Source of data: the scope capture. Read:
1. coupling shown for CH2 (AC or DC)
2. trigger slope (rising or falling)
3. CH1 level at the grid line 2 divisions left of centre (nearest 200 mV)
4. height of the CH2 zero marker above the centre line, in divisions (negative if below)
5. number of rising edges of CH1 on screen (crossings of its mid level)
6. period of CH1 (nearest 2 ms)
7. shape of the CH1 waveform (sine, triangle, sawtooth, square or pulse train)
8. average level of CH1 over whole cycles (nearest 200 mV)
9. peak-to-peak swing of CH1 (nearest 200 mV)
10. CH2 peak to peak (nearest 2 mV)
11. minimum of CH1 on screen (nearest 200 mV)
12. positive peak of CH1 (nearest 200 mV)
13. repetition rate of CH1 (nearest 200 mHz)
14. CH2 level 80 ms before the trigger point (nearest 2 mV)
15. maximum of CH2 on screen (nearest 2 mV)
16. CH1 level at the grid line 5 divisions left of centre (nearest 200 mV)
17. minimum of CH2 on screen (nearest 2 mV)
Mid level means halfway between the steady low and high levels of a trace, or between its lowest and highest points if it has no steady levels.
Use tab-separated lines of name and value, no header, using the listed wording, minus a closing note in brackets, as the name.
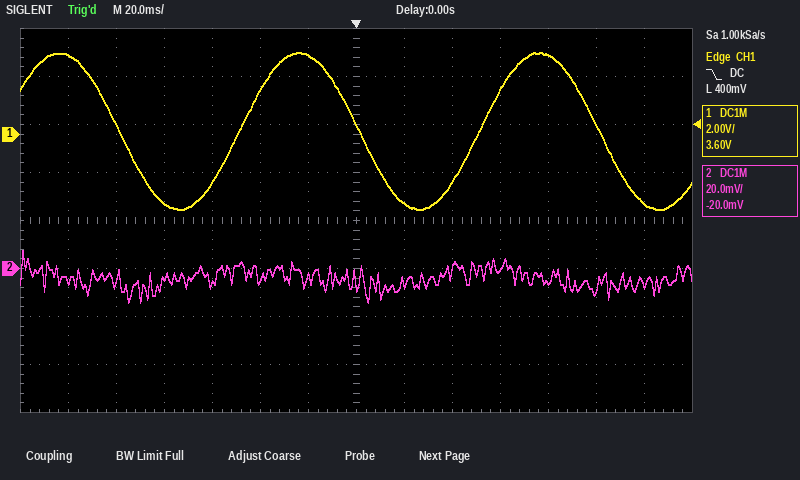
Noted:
coupling shown for CH2	DC
trigger slope	falling
CH1 level at the grid line 2 divisions left of centre	1.8 V
height of the CH2 zero marker above the centre line, in divisions	-1.0 div
number of rising edges of CH1 on screen	2
period of CH1	100 ms
shape of the CH1 waveform	sine
average level of CH1 over whole cycles	200 mV
peak-to-peak swing of CH1	6.6 V
CH2 peak to peak	22 mV
minimum of CH1 on screen	-3.2 V
positive peak of CH1	3.4 V
repetition rate of CH1	10.0 Hz
CH2 level 80 ms before the trigger point	-4 mV
maximum of CH2 on screen	8 mV
CH1 level at the grid line 5 divisions left of centre	400 mV
minimum of CH2 on screen	-14 mV
